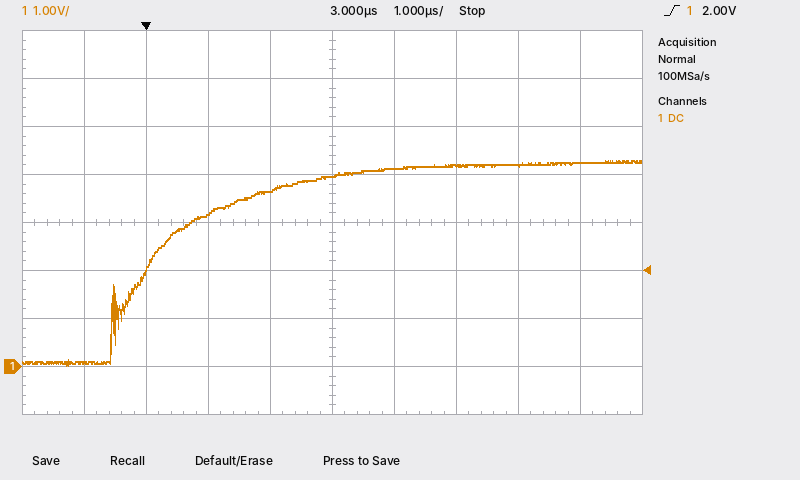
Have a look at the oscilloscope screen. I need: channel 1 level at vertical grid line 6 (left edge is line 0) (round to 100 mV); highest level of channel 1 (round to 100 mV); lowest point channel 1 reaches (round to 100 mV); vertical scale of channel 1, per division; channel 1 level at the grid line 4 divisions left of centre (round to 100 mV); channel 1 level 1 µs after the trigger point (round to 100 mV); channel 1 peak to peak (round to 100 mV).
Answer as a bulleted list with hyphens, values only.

- 4.1 V
- 4.3 V
- 0.0 V
- 1 V
- 100 mV
- 3.2 V
- 4.3 V
